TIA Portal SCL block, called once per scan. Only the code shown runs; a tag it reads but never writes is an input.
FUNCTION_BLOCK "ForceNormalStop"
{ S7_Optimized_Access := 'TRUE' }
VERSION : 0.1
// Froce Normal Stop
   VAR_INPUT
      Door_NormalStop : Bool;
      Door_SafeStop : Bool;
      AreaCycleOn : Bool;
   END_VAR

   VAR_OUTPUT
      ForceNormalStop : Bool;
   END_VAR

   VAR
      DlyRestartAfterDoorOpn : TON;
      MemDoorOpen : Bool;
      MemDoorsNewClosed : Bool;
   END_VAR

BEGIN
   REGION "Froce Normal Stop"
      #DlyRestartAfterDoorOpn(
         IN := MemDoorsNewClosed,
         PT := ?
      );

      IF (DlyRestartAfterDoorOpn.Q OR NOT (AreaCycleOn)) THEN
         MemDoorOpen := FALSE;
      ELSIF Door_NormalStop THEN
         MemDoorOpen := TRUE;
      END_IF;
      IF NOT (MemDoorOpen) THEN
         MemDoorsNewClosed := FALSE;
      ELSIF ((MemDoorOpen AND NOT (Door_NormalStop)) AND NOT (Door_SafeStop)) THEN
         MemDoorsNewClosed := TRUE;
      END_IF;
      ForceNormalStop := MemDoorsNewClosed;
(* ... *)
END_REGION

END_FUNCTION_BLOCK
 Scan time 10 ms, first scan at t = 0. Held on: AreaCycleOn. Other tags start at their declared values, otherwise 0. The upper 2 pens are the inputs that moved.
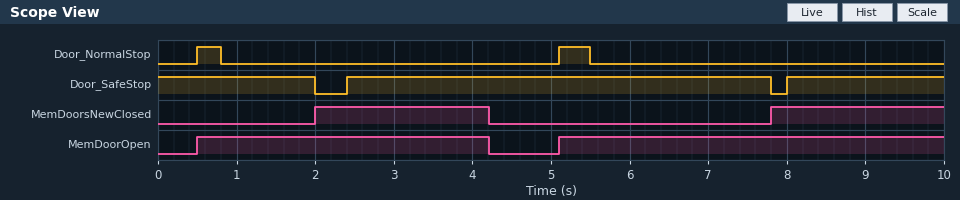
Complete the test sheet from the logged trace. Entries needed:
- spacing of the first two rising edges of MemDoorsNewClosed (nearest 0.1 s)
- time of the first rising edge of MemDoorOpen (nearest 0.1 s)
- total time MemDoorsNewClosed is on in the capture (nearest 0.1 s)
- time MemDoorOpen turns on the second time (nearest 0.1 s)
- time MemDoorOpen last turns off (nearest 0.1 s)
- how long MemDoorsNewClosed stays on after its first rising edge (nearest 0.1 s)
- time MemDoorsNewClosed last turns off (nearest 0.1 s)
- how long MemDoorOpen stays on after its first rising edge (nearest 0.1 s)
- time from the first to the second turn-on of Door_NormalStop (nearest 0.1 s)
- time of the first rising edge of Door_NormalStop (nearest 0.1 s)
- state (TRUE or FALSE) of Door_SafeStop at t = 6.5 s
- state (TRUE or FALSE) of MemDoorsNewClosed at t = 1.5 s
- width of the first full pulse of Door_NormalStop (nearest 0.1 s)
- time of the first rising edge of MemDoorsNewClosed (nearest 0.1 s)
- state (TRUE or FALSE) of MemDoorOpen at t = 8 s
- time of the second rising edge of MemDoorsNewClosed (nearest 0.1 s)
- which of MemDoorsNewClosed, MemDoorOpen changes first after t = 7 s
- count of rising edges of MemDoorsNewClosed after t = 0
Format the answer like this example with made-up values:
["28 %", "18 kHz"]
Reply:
["5.8 s", "0.5 s", "4.4 s", "5.1 s", "4.2 s", "2.2 s", "4.2 s", "3.7 s", "4.6 s", "0.5 s", "TRUE", "FALSE", "0.3 s", "2.0 s", "TRUE", "7.8 s", "MemDoorsNewClosed", "2"]
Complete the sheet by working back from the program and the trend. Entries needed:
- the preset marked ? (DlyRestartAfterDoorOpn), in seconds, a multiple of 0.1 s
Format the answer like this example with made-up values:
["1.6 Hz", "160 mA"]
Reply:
["2.2 s"]
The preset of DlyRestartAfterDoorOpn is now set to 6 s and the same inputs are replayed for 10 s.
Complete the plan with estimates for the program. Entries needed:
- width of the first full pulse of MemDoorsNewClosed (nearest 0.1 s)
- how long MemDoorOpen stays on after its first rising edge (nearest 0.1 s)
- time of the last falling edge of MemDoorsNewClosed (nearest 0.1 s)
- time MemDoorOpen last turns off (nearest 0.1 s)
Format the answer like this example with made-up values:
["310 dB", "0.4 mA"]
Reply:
["6.0 s", "7.5 s", "8.0 s", "8.0 s"]
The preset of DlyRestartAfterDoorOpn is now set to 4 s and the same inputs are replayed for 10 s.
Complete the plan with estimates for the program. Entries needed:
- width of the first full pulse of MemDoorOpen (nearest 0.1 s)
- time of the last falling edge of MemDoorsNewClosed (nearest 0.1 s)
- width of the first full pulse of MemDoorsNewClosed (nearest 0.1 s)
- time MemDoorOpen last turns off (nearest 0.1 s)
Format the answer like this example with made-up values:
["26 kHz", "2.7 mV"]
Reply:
["5.5 s", "6.0 s", "4.0 s", "6.0 s"]
